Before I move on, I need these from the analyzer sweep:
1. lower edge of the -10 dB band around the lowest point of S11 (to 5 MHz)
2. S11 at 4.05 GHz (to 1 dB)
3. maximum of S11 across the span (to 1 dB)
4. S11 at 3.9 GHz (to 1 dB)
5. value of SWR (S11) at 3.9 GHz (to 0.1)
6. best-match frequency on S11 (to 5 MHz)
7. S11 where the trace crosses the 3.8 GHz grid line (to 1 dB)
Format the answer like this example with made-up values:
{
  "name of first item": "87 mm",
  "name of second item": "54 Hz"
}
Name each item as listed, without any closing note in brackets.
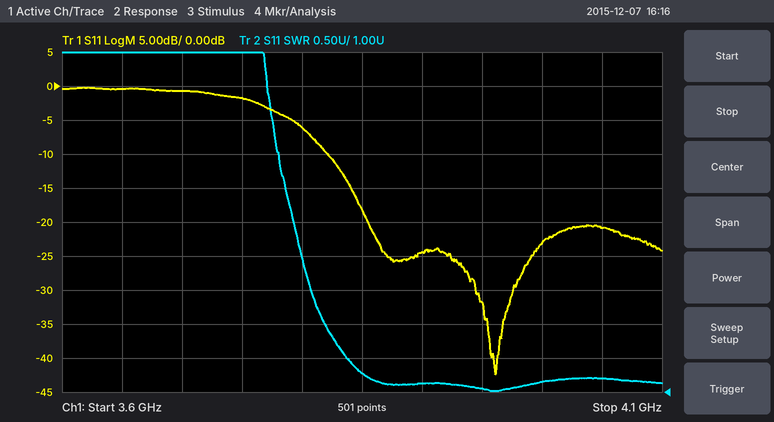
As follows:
{
  "lower edge of the -10 dB band around the lowest point of S11": "3.820 GHz",
  "S11 at 4.05 GHz": "-21 dB",
  "maximum of S11 across the span": "0 dB",
  "S11 at 3.9 GHz": "-24 dB",
  "value of SWR (S11) at 3.9 GHz": "1.1",
  "best-match frequency on S11": "3.960 GHz",
  "S11 where the trace crosses the 3.8 GHz grid line": "-6 dB"
}
